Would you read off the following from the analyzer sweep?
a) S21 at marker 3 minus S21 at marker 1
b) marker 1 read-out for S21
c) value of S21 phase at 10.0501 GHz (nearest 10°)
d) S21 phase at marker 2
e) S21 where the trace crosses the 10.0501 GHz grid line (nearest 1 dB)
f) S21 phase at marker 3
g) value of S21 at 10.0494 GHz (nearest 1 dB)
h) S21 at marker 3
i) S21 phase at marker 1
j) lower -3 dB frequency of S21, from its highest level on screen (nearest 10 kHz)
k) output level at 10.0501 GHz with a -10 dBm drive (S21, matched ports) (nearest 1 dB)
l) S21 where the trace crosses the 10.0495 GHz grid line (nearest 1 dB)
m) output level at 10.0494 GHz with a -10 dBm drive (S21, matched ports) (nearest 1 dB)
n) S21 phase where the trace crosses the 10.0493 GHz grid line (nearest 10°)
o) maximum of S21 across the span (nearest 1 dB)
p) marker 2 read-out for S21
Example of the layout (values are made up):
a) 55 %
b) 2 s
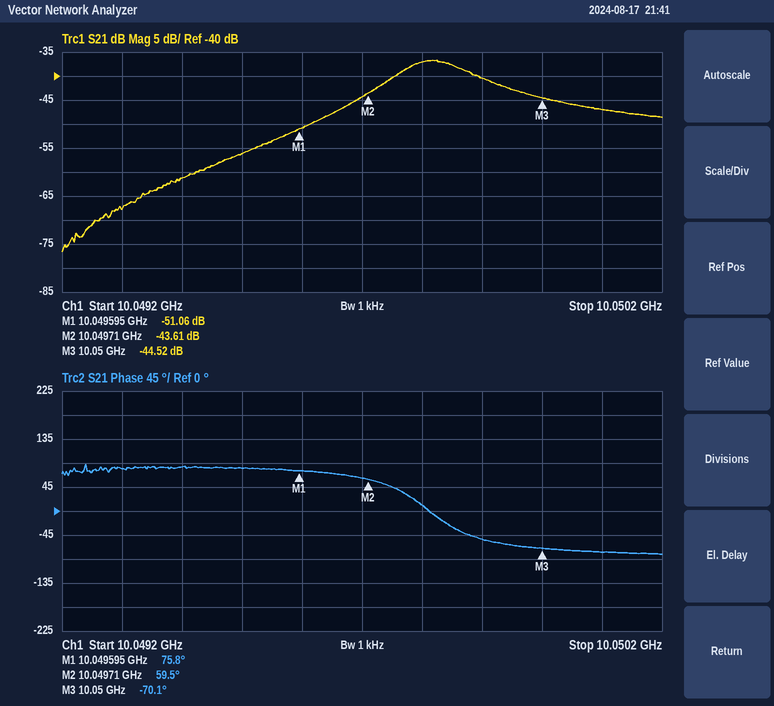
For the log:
a) 6.54 dB
b) -51.06 dB
c) -80°
d) 59.5°
e) -47 dB
f) -70.1°
g) -61 dB
h) -44.52 dB
i) 75.8°
j) 10.04976 GHz
k) -57 dBm
l) -56 dB
m) -71 dBm
n) 80°
o) -37 dB
p) -43.61 dB
